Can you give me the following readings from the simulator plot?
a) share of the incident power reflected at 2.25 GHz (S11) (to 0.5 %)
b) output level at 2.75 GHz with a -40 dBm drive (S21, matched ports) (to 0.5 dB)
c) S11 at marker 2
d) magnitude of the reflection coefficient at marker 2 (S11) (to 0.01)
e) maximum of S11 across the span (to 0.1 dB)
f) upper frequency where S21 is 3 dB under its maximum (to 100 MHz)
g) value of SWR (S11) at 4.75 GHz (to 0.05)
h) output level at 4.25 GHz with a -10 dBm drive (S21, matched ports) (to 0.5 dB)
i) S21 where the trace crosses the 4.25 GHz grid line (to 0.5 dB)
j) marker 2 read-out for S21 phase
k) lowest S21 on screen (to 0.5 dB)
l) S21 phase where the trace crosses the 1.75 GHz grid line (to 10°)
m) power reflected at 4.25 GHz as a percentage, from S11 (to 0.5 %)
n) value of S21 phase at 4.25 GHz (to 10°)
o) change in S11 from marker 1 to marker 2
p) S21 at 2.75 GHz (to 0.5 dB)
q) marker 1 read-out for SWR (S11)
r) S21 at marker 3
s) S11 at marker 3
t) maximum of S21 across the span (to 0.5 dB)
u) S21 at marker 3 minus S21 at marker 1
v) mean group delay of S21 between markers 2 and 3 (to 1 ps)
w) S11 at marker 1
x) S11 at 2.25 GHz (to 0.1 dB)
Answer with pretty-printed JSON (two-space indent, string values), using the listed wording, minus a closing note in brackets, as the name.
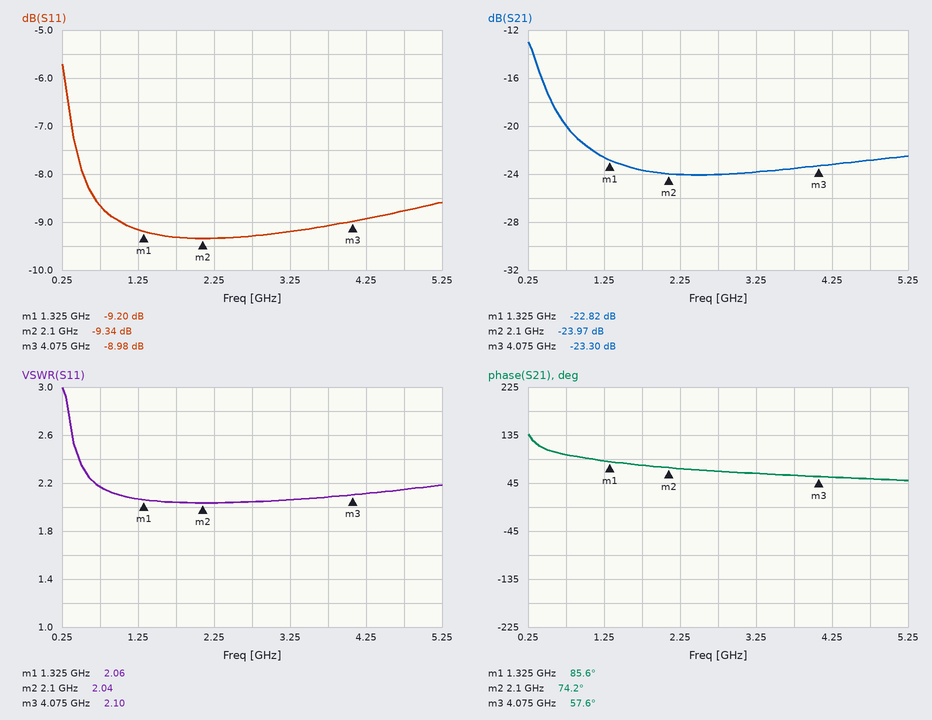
{
  "share of the incident power reflected at 2.25 GHz (S11)": "11.5 %",
  "output level at 2.75 GHz with a -40 dBm drive (S21, matched ports)": "-64.0 dBm",
  "S11 at marker 2": "-9.34 dB",
  "magnitude of the reflection coefficient at marker 2 (S11)": "0.34",
  "maximum of S11 across the span": "-5.7 dB",
  "upper frequency where S21 is 3 dB under its maximum": "400 MHz",
  "value of SWR (S11) at 4.75 GHz": "2.15",
  "output level at 4.25 GHz with a -10 dBm drive (S21, matched ports)": "-33.0 dBm",
  "S21 where the trace crosses the 4.25 GHz grid line": "-23.0 dB",
  "marker 2 read-out for S21 phase": "74.2°",
  "lowest S21 on screen": "-24.0 dB",
  "S21 phase where the trace crosses the 1.75 GHz grid line": "80°",
  "power reflected at 4.25 GHz as a percentage, from S11": "13.0 %",
  "value of S21 phase at 4.25 GHz": "60°",
  "change in S11 from marker 1 to marker 2": "-0.14 dB",
  "S21 at 2.75 GHz": "-24.0 dB",
  "marker 1 read-out for SWR": "2.06",
  "S21 at marker 3": "-23.30 dB",
  "S11 at marker 3": "-8.98 dB",
  "maximum of S21 across the span": "-13.0 dB",
  "S21 at marker 3 minus S21 at marker 1": "-0.48 dB",
  "mean group delay of S21 between markers 2 and 3": "23 ps",
  "S11 at marker 1": "-9.20 dB",
  "S11 at 2.25 GHz": "-9.3 dB"
}
